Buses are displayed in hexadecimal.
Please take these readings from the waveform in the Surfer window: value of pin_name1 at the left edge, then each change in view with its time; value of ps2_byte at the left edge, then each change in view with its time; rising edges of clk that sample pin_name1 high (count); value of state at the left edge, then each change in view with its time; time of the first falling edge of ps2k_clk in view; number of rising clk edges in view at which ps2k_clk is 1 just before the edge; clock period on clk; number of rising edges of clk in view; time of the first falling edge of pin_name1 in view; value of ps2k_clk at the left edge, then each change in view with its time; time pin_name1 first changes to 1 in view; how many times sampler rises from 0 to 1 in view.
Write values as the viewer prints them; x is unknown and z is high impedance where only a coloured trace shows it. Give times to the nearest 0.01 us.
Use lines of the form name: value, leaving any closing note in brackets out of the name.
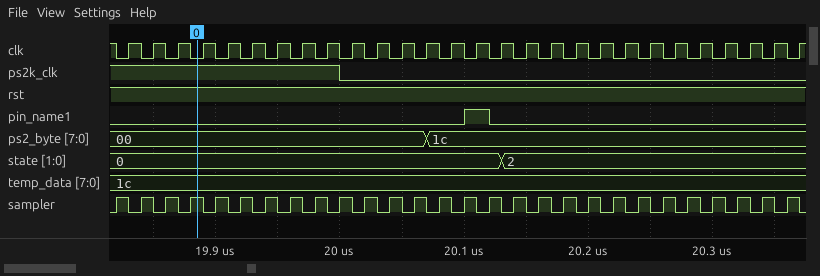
value of pin_name1 at the left edge, then each change in view with its time: 0, 1 at 20.1 us, 0 at 20.12 us
value of ps2_byte at the left edge, then each change in view with its time: 00, 1c at 20.07 us
rising edges of clk that sample pin_name1 high: 1
value of state at the left edge, then each change in view with its time: 0, 2 at 20.13 us
time of the first falling edge of ps2k_clk in view: 20 us
number of rising clk edges in view at which ps2k_clk is 1 just before the edge: 9
clock period on clk: 0.02 us
number of rising edges of clk in view: 28
time of the first falling edge of pin_name1 in view: 20.12 us
value of ps2k_clk at the left edge, then each change in view with its time: 1, 0 at 20 us
time pin_name1 first changes to 1 in view: 20.1 us
how many times sampler rises from 0 to 1 in view: 28
